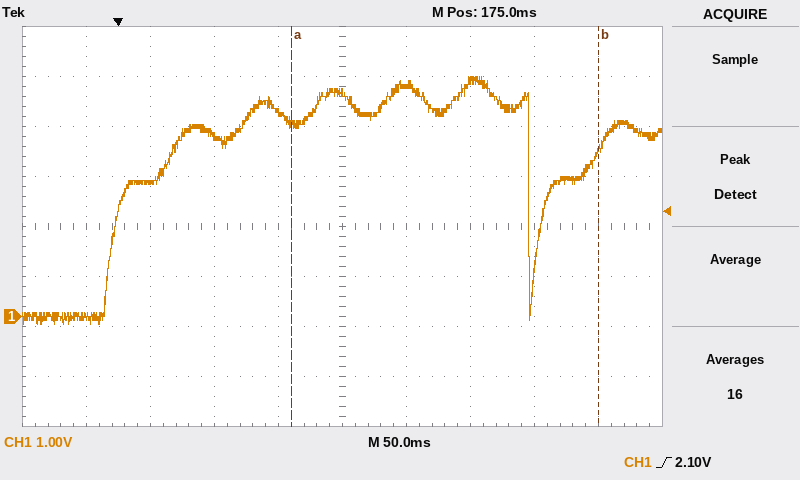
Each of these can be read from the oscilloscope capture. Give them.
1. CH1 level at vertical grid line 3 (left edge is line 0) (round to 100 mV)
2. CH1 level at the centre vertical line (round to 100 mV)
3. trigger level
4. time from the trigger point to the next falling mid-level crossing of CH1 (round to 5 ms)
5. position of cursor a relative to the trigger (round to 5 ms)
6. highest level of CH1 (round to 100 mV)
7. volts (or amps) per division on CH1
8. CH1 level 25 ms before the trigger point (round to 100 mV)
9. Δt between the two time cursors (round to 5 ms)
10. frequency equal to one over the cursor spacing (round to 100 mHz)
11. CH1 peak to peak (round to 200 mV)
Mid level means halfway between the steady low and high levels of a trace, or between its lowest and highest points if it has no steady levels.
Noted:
3.6 V
4.5 V
2.10 V
320 ms
+135 ms
4.8 V
1 V
0.0 V
240 ms
4.2 Hz
5.0 V
